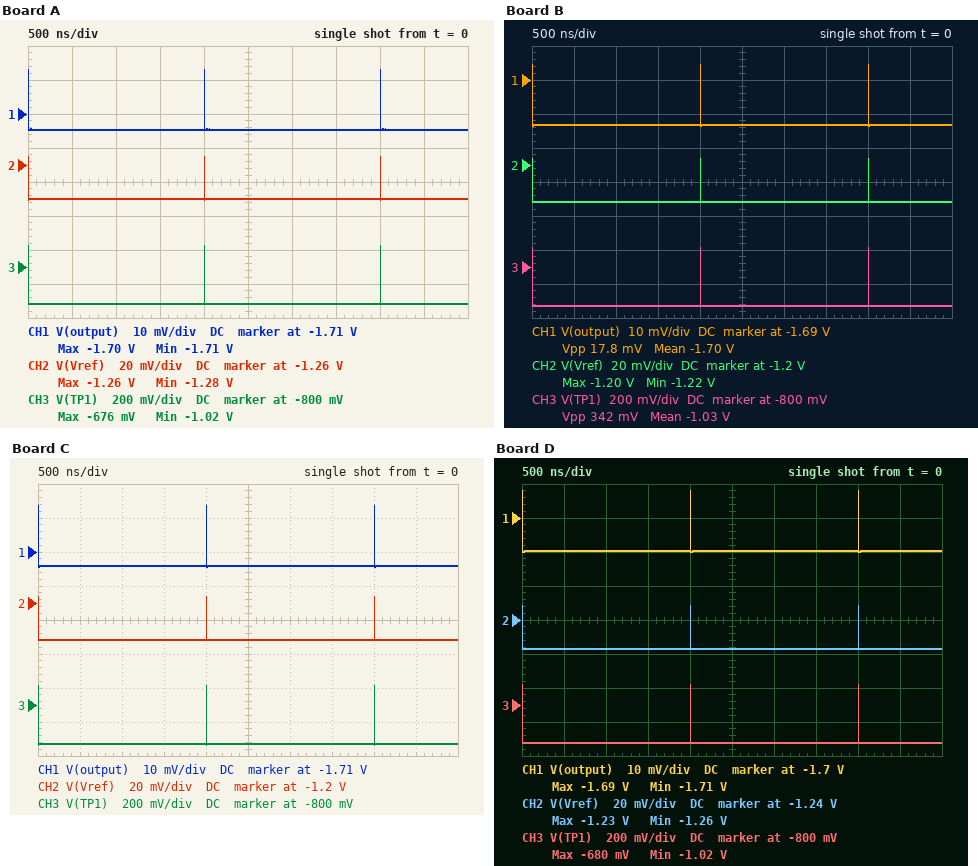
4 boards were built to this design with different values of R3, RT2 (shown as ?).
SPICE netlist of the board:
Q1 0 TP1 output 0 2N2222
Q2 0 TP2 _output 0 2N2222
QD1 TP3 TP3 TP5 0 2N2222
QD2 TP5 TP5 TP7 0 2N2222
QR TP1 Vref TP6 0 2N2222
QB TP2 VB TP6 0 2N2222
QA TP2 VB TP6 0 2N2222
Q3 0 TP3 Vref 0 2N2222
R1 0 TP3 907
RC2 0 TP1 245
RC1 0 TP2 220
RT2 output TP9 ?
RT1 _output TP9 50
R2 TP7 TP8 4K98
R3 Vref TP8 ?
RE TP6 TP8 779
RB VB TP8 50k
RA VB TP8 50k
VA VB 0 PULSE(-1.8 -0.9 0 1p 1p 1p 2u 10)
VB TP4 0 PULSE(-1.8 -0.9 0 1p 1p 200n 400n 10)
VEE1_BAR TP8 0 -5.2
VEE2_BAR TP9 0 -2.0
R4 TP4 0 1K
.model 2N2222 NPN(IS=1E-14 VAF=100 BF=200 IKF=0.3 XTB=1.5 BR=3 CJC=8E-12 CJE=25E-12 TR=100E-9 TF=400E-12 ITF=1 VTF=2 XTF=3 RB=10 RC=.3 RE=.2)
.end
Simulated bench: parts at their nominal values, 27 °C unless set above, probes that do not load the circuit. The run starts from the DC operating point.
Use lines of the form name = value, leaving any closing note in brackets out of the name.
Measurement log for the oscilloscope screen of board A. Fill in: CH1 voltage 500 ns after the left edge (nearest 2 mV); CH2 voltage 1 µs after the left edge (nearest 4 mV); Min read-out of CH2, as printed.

CH1 voltage 500 ns after the left edge = -1.714 V
CH2 voltage 1 µs after the left edge = -1.280 V
Min read-out of CH2, as printed = -1.28 V
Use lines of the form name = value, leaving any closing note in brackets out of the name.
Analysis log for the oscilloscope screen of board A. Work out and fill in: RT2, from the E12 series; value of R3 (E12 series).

RT2, from the E12 series = 56 Ω
value of R3 = 2.2 kΩ
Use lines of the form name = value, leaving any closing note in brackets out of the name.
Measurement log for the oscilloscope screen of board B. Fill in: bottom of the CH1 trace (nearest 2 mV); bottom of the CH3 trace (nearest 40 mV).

bottom of the CH1 trace = -1.704 V
bottom of the CH3 trace = -1.04 V
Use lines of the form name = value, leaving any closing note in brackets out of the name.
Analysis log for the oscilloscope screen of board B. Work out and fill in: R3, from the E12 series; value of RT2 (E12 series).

R3, from the E12 series = 18 kΩ
value of RT2 = 150 Ω
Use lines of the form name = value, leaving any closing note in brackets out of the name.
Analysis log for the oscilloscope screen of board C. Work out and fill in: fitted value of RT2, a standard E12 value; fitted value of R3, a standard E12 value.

fitted value of RT2, a standard E12 value = 100 Ω
fitted value of R3, a standard E12 value = 18 kΩ
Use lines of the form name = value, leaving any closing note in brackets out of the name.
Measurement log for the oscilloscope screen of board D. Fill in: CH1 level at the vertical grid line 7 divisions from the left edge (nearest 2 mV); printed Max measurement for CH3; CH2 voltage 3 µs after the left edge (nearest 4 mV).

CH1 level at the vertical grid line 7 divisions from the left edge = -1.710 V
printed Max measurement for CH3 = -680 mV
CH2 voltage 3 µs after the left edge = -1.256 V
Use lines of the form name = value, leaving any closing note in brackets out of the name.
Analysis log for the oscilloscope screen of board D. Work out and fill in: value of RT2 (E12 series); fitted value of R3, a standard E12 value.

value of RT2 = 82 Ω
fitted value of R3, a standard E12 value = 4.7 kΩ
